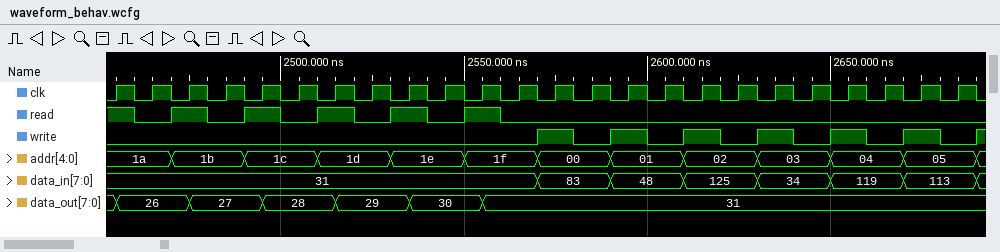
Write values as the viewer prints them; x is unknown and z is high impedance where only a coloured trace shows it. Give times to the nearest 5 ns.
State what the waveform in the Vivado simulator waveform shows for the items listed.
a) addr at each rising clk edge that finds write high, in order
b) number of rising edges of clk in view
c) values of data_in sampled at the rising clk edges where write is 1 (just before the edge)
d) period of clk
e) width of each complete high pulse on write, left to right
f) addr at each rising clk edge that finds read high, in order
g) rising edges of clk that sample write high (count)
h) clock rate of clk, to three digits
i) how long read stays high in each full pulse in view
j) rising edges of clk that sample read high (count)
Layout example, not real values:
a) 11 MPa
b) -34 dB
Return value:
a) 00, 01, 02, 03, 04, 05
b) 24
c) 83, 48, 125, 34, 119, 113
d) 10 ns
e) 10 ns, 10 ns, 10 ns, 10 ns, 10 ns, 10 ns
f) 1a, 1b, 1c, 1d, 1e, 1f
g) 6
h) 100 MHz
i) 10 ns, 10 ns, 10 ns, 10 ns, 10 ns
j) 6
